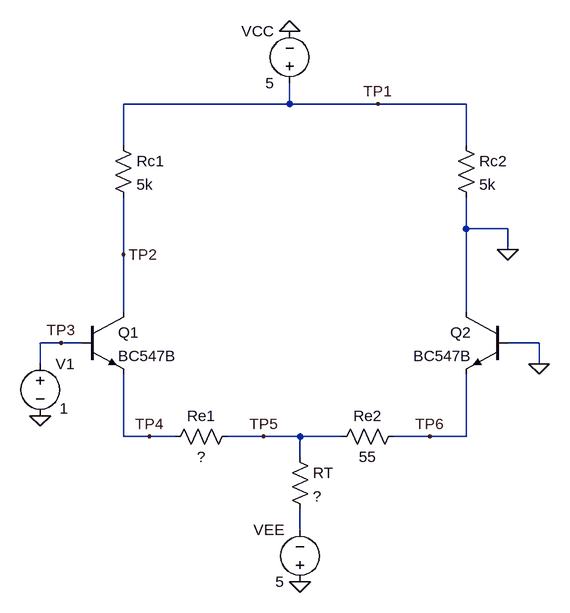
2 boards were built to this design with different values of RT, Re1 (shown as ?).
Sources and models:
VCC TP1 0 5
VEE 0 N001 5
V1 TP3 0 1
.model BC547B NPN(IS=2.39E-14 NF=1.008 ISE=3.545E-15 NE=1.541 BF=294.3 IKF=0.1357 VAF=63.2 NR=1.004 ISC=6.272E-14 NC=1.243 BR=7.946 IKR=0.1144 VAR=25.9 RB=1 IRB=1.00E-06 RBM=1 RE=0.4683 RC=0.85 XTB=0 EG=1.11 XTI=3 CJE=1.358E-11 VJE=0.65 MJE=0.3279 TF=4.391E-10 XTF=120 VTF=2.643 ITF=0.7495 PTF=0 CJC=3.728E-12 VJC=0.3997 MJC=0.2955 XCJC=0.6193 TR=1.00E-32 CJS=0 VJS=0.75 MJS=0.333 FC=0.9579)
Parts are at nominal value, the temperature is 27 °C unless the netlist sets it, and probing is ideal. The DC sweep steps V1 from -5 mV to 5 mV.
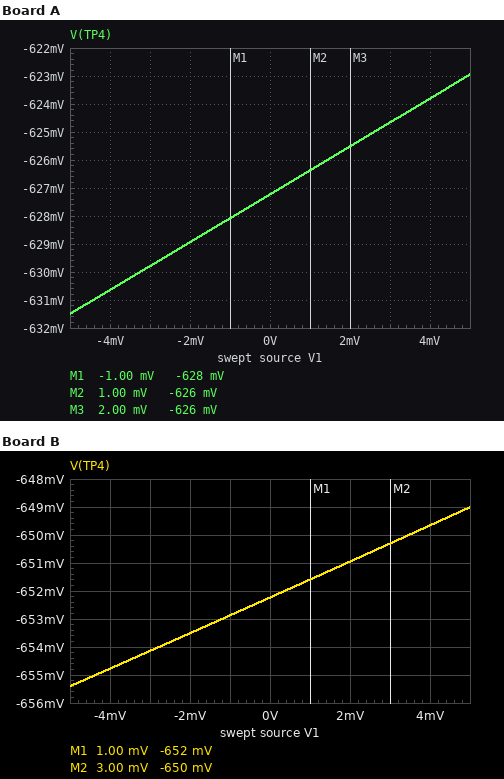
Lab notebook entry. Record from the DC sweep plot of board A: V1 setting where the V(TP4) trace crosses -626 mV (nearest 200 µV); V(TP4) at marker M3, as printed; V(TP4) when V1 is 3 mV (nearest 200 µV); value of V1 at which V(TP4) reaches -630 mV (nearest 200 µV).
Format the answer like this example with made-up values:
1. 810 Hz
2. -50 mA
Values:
1. 1.4 mV
2. -626 mV
3. -624.6 mV
4. -3.2 mV
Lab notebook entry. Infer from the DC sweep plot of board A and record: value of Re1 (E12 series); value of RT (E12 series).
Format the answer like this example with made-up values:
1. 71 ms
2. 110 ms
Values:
1. 180 Ω
2. 1.8 kΩ
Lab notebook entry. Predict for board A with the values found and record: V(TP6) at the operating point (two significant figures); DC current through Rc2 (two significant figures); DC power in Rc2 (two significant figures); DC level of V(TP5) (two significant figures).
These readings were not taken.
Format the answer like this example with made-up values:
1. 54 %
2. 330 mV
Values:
1. -190 mV
2. 1.0 mA
3. 5.0 mW
4. -190 mV
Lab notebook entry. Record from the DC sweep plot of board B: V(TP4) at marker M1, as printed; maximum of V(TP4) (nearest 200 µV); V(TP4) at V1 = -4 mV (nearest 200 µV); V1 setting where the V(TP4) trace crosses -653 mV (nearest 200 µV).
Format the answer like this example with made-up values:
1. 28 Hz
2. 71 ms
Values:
1. -652 mV
2. -649.0 mV
3. -654.8 mV
4. -1.2 mV
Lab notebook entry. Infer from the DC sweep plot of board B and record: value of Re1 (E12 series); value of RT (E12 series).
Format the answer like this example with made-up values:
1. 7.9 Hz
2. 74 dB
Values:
1. 150 Ω
2. 1 kΩ
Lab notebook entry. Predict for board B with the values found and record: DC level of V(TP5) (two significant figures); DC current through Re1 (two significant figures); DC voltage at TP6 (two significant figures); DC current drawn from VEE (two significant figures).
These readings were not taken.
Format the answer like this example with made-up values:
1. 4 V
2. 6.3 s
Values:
1. -420 mV
2. 4.6 mA
3. -420 mV
4. 4.6 mA
